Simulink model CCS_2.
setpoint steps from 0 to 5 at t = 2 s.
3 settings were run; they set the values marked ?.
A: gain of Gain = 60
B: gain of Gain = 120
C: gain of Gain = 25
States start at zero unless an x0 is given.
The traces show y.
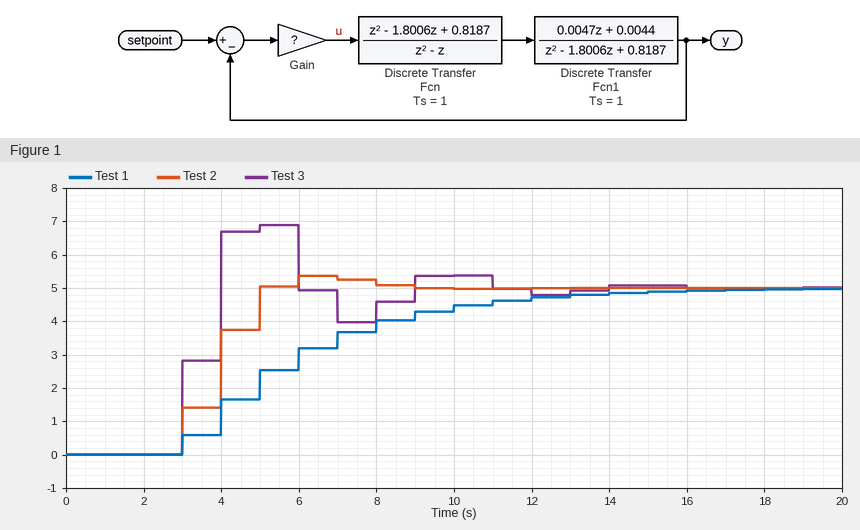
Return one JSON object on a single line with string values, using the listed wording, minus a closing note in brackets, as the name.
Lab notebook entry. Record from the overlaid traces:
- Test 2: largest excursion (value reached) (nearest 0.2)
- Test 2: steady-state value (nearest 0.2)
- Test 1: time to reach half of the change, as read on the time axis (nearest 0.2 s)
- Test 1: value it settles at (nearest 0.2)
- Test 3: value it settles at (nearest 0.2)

{"Test 2: largest excursion (value reached)": "5.4", "Test 2: steady-state value": "5.0", "Test 1: time to reach half of the change, as read on the time axis": "5.0 s", "Test 1: value it settles at": "5.0", "Test 3: value it settles at": "5.0"}
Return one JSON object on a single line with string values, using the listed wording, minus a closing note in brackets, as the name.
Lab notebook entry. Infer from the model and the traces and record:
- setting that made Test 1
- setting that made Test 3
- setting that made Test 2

{"setting that made Test 1": "C", "setting that made Test 3": "B", "setting that made Test 2": "A"}
